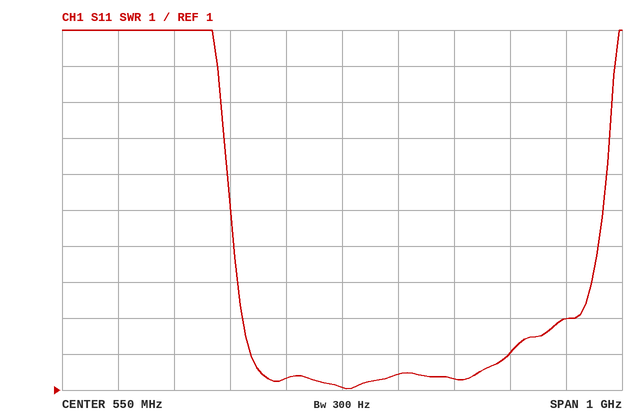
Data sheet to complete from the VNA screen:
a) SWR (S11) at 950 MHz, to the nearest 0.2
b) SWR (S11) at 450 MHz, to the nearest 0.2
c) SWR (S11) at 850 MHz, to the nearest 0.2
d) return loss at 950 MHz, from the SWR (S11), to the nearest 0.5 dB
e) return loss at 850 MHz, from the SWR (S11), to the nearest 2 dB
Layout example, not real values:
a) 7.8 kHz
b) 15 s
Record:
a) 3.0
b) 1.4
c) 2.0
d) 6.0 dB
e) 10 dB
